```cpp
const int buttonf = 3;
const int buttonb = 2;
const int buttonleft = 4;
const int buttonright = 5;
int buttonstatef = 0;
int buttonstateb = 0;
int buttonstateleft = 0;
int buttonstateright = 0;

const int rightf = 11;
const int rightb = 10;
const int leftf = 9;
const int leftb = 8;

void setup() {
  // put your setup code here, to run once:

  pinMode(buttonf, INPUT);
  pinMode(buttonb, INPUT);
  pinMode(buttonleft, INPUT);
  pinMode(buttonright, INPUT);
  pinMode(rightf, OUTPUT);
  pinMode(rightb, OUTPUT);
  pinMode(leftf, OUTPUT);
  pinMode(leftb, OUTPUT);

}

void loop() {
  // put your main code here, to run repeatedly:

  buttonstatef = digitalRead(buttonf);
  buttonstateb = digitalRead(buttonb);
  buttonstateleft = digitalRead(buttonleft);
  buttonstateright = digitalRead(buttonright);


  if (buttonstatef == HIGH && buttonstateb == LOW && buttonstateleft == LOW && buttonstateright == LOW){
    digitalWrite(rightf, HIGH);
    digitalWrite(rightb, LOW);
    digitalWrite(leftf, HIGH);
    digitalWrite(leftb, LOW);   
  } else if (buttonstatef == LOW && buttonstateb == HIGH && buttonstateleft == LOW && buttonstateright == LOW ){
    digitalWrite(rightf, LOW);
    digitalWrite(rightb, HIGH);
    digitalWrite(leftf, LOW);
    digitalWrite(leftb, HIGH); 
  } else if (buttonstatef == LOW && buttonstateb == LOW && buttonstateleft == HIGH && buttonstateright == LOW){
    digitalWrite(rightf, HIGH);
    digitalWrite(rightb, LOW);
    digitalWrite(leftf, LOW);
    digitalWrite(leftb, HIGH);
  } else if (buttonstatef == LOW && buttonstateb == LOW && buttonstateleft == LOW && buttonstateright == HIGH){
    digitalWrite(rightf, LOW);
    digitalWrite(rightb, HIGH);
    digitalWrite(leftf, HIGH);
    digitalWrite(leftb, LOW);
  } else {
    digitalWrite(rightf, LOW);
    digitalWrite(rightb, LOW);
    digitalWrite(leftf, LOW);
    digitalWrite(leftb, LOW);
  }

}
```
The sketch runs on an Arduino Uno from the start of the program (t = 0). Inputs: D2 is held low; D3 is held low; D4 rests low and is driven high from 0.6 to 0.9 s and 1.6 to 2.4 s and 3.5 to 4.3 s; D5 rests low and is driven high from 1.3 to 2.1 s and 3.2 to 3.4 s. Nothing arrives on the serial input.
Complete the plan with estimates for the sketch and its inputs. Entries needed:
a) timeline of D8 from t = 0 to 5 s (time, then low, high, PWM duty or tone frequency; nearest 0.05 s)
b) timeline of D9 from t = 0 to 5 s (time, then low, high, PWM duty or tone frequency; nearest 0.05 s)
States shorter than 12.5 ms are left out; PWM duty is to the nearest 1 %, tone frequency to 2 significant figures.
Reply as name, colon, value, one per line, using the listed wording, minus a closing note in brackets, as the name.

timeline of D8 from t = 0 to 5 s: 0 s low; 0.6 s high; 0.9 s low; 2.1 s high; 2.4 s low; 3.5 s high; 4.3 s low
timeline of D9 from t = 0 to 5 s: 0 s low; 1.3 s high; 1.6 s low; 3.2 s high; 3.4 s low
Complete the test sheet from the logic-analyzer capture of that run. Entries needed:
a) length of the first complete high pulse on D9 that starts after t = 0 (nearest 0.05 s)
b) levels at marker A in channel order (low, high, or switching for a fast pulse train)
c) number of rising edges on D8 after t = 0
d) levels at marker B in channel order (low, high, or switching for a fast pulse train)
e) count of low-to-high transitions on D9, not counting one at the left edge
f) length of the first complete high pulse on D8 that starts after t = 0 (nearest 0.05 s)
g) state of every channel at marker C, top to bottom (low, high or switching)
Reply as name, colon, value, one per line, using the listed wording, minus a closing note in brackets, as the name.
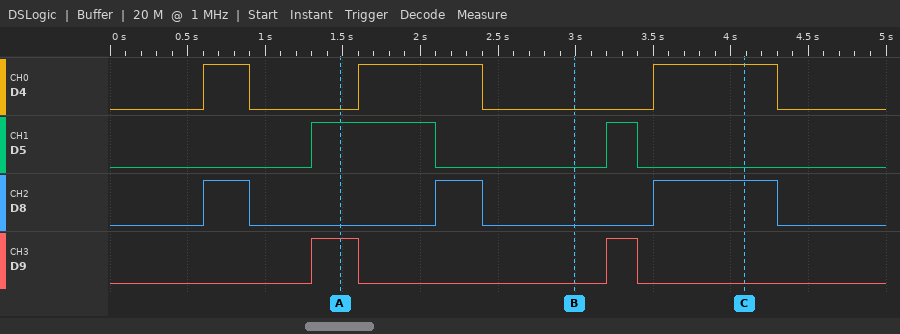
length of the first complete high pulse on D9 that starts after t = 0: 0.30 s
levels at marker A in channel order: D4 low, D5 high, D8 low, D9 high
number of rising edges on D8 after t = 0: 3
levels at marker B in channel order: D4 low, D5 low, D8 low, D9 low
count of low-to-high transitions on D9, not counting one at the left edge: 2
length of the first complete high pulse on D8 that starts after t = 0: 0.30 s
state of every channel at marker C, top to bottom: D4 high, D5 low, D8 high, D9 low
